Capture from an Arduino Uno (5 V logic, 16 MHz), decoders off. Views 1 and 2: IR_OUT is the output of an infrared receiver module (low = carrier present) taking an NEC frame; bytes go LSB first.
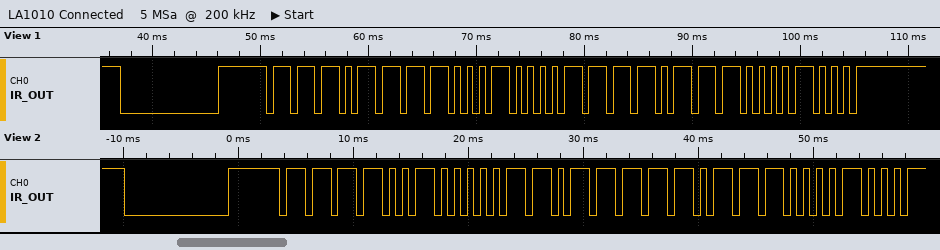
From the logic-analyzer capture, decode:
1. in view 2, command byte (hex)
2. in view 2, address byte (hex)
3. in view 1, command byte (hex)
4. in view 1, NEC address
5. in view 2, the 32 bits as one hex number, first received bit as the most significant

0xEF
0x4F
0xEF
0xF7
0xF20DF708
